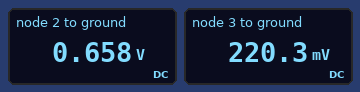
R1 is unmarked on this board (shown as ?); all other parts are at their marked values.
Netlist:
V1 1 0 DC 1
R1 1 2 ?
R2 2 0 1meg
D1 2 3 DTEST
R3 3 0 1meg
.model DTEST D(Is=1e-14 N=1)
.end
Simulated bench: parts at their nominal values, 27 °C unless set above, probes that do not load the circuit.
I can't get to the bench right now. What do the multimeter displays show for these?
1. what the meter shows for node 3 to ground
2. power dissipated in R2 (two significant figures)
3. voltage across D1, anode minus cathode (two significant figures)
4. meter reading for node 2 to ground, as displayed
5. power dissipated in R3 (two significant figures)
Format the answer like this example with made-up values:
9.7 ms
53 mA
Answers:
220.3 mV
430 nW
440 mV
0.658 V
49 nW
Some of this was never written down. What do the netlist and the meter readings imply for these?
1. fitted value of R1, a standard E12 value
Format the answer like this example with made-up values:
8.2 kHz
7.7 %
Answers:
390 kΩ
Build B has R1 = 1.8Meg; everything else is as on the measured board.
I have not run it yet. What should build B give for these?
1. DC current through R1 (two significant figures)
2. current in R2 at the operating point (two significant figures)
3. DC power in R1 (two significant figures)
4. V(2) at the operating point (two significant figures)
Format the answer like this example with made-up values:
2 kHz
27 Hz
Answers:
360 nA
350 nA
230 nW
350 mV
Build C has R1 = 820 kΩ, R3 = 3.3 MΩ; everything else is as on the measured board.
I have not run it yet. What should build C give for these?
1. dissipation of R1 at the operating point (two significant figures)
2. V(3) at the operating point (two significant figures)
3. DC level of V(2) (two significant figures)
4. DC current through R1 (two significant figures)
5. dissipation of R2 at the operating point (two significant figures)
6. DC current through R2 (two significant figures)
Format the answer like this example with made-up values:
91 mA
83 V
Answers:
270 nW
140 mV
530 mV
570 nA
280 nW
530 nA
